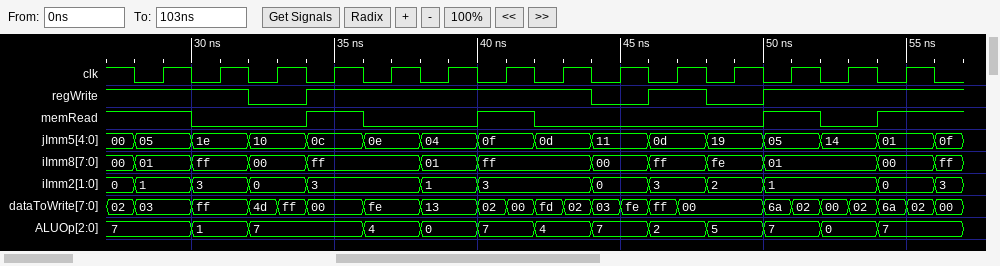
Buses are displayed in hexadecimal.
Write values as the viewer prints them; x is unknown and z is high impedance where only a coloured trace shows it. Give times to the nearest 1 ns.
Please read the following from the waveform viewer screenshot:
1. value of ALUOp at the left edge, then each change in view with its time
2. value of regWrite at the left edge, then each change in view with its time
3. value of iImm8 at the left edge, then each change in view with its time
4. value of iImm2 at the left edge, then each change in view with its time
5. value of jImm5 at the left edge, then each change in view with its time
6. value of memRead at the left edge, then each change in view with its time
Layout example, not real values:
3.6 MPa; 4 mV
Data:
7, 1 at 30 ns, 7 at 32 ns, 4 at 36 ns, 0 at 38 ns, 7 at 40 ns, 4 at 42 ns, 7 at 44 ns, 2 at 46 ns, 5 at 48 ns, 7 at 50 ns, 0 at 52 ns, 7 at 54 ns; 1, 0 at 32 ns, 1 at 34 ns, 0 at 44 ns, 1 at 46 ns, 0 at 48 ns, 1 at 50 ns; 00, 01 at 28 ns, ff at 30 ns, 00 at 32 ns, ff at 34 ns, 01 at 38 ns, ff at 40 ns, 00 at 44 ns, ff at 46 ns, fe at 48 ns, 01 at 50 ns, 00 at 54 ns, ff at 56 ns; 0, 1 at 28 ns, 3 at 30 ns, 0 at 32 ns, 3 at 34 ns, 1 at 38 ns, 3 at 40 ns, 0 at 44 ns, 3 at 46 ns, 2 at 48 ns, 1 at 50 ns, 0 at 54 ns, 3 at 56 ns; 00, 05 at 28 ns, 1e at 30 ns, 10 at 32 ns, 0c at 34 ns, 0e at 36 ns, 04 at 38 ns, 0f at 40 ns, 0d at 42 ns, 11 at 44 ns, 0d at 46 ns, 19 at 48 ns, 05 at 50 ns, 14 at 52 ns, 01 at 54 ns, 0f at 56 ns; 1, 0 at 30 ns, 1 at 34 ns, 0 at 36 ns, 1 at 40 ns, 0 at 42 ns, 1 at 50 ns, 0 at 52 ns, 1 at 54 ns
